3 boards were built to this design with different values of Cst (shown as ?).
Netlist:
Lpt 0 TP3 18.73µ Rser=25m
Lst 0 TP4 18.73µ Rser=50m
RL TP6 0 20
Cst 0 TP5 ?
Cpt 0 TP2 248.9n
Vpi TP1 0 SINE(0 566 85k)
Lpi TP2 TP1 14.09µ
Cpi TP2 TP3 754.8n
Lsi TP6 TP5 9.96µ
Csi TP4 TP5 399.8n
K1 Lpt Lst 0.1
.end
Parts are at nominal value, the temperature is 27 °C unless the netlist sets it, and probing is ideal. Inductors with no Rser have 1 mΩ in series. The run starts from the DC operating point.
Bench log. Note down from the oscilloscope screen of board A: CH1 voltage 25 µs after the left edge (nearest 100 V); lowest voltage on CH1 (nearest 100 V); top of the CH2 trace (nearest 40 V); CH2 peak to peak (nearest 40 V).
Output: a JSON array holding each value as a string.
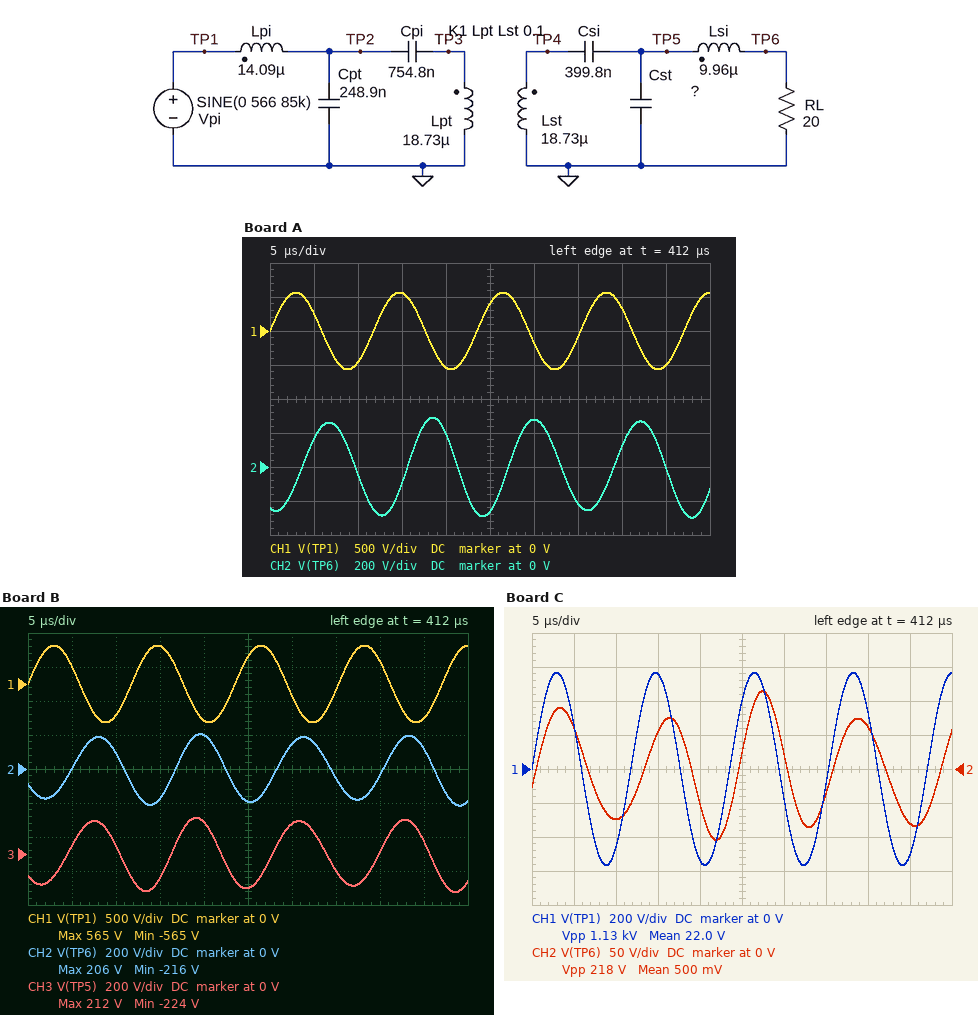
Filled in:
["400 V", "-600 V", "280 V", "600 V"]
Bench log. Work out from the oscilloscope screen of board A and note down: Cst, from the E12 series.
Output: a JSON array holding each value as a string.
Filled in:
["390 nF"]
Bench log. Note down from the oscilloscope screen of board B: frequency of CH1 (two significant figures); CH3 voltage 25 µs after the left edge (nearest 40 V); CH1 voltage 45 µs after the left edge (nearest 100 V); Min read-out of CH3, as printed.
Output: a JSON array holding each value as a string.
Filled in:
["85 kHz", "-200 V", "-500 V", "-224 V"]
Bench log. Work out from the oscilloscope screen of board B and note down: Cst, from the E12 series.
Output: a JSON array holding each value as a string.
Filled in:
["470 nF"]
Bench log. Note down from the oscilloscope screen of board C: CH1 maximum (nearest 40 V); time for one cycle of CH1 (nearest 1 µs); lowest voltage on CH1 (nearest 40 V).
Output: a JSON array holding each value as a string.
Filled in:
["560 V", "12 µs", "-560 V"]
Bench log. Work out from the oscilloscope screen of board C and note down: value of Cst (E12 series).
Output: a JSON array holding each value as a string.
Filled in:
["100 nF"]
